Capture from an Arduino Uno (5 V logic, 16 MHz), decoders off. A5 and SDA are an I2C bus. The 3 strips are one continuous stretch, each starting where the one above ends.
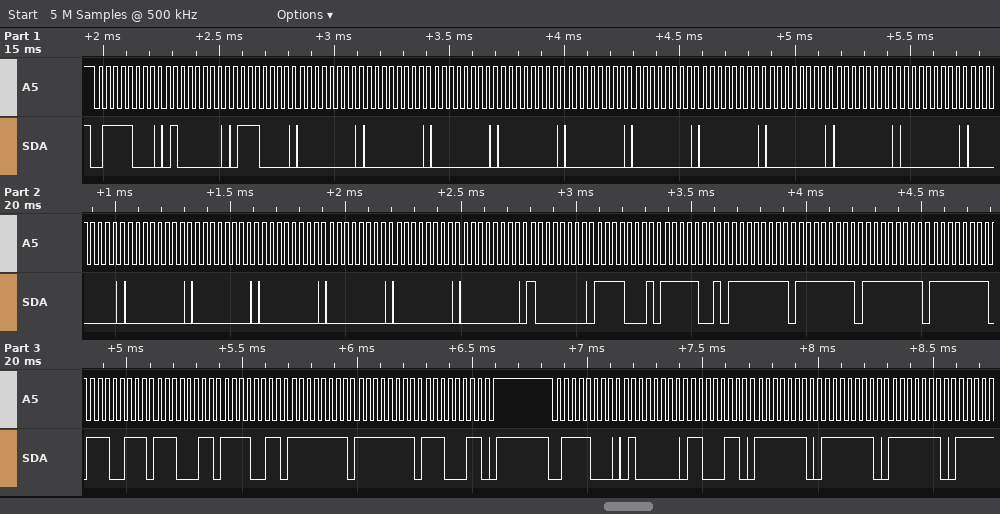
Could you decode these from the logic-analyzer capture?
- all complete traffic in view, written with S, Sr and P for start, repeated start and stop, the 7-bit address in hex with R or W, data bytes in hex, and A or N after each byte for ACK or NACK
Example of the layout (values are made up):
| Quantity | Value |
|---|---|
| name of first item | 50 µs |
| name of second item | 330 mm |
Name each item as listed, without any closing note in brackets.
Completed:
| Quantity | Value |
|---|---|
| all complete traffic in view, written with S, Sr and P for start, repeated start and stop, the 7-bit address in hex with R or W, data bytes in hex, and A or N after each byte for ACK or NACK | S 3CW A 40 A 70 A 00 A 00 A 00 A 00 A 00 A 00 A 00 A 00 A 00 A 00 A 00 A 00 A 00 A 00 A 00 A 00 A 00 A 80 A F1 A F9 A FF A FF A FF A FF A E7 A E3 A F3 A FF A FF A E3 A P S 3CW A 40 A C6 A FE A FE A FE A |
